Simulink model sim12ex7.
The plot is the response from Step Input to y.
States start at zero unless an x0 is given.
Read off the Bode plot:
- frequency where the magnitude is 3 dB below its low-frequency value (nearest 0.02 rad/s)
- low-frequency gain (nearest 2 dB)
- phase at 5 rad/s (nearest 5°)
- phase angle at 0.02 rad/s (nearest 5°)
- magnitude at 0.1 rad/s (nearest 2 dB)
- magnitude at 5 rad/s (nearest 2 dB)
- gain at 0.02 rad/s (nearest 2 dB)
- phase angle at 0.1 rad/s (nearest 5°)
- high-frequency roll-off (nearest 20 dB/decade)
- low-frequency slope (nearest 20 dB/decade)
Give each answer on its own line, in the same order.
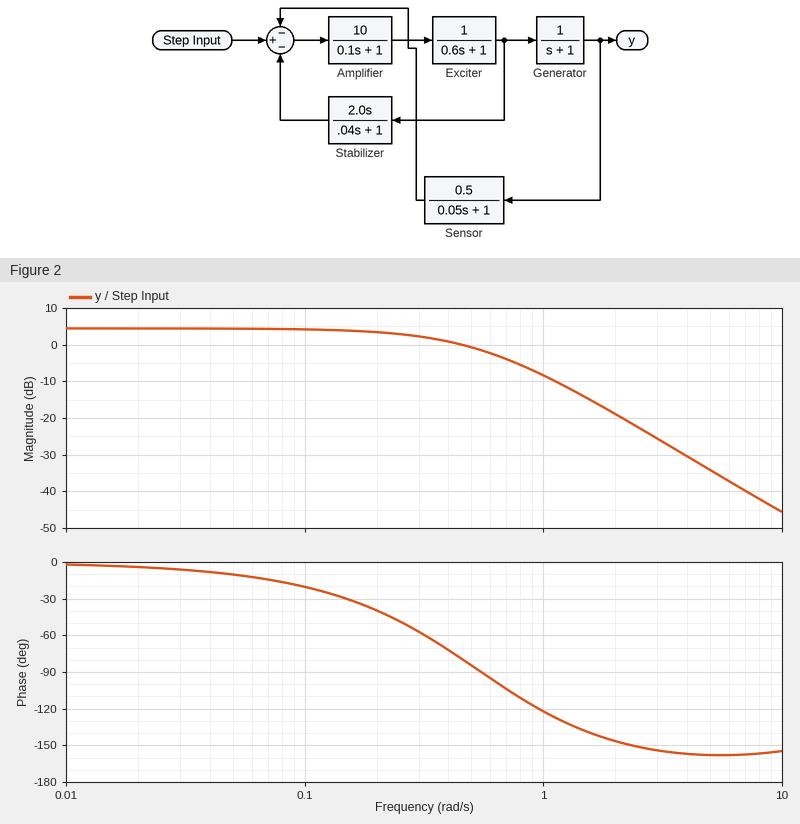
0.36 rad/s
4 dB
-160°
-5°
4 dB
-34 dB
4 dB
-20°
-40 dB/decade
0 dB/decade
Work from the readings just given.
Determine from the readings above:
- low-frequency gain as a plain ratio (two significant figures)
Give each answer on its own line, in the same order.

1.6
